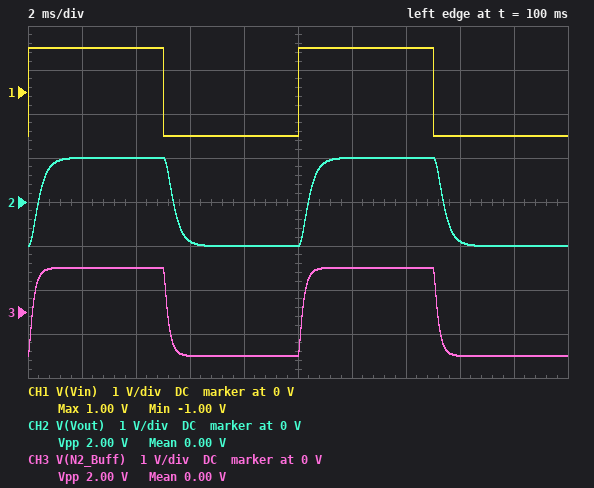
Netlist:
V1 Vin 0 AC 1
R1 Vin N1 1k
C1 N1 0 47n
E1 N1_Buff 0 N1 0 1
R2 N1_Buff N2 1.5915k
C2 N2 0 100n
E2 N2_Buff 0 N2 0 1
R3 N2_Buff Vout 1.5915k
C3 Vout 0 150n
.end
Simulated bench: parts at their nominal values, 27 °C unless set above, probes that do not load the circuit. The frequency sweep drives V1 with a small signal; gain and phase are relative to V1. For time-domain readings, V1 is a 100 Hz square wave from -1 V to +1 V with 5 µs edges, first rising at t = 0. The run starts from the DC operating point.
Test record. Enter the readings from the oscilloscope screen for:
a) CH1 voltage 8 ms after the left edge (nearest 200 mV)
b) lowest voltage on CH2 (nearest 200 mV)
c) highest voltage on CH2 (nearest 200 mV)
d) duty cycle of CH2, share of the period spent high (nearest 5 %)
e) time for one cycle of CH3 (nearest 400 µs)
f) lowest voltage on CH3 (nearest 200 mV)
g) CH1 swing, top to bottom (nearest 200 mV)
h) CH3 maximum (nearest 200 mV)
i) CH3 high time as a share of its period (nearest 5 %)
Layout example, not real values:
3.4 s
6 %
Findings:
-1.0 V
-1.0 V
1.0 V
50 %
10.0 ms
-1.0 V
2.0 V
1.0 V
50 %
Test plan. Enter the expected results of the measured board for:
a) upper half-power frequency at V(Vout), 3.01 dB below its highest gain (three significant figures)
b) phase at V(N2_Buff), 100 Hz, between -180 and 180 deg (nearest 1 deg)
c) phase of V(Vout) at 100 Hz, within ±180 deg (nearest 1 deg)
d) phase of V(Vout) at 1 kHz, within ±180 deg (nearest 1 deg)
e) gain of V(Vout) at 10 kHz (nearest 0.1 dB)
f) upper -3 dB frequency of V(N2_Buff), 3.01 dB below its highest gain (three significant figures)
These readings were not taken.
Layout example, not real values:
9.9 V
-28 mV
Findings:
501 Hz
-7 deg
-16 deg
-118 deg
-53.5 dB
928 Hz
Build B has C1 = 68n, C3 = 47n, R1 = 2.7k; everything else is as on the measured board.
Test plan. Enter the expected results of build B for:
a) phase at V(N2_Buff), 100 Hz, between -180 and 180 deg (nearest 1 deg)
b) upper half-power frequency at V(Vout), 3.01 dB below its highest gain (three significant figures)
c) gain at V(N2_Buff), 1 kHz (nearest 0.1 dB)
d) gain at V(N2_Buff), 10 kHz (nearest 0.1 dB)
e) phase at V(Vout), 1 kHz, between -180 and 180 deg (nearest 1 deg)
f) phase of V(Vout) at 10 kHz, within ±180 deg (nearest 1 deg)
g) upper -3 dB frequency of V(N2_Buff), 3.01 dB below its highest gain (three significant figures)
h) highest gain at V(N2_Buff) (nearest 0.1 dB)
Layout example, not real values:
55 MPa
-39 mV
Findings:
-12 deg
562 Hz
-6.7 dB
-41.3 dB
-119 deg
113 deg
597 Hz
0 dB
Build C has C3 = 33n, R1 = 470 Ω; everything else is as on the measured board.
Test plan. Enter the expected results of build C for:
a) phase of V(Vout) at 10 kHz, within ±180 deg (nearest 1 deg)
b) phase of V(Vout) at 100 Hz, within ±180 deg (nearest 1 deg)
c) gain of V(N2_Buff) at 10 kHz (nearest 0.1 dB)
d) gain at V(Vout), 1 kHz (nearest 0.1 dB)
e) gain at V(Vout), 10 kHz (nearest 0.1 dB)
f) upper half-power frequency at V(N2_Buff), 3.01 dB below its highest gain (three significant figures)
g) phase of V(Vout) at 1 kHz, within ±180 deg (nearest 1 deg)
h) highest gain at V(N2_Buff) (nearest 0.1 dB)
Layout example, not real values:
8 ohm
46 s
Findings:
148 deg
-8 deg
-24.7 dB
-3.5 dB
-35.5 dB
982 Hz
-71 deg
0 dB
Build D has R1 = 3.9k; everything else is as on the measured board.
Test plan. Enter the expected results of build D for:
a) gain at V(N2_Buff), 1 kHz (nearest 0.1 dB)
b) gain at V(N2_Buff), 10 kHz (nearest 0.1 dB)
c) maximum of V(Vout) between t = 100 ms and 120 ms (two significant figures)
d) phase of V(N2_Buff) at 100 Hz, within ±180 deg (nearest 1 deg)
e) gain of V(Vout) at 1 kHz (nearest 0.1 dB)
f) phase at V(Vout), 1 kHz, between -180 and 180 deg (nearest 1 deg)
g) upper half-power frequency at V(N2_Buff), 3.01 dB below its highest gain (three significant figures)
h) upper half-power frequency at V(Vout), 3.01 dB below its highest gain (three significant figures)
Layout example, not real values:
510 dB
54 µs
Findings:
-6.7 dB
-41.3 dB
1.0 V
-12 deg
-11.8 dB
-150 deg
598 Hz
415 Hz
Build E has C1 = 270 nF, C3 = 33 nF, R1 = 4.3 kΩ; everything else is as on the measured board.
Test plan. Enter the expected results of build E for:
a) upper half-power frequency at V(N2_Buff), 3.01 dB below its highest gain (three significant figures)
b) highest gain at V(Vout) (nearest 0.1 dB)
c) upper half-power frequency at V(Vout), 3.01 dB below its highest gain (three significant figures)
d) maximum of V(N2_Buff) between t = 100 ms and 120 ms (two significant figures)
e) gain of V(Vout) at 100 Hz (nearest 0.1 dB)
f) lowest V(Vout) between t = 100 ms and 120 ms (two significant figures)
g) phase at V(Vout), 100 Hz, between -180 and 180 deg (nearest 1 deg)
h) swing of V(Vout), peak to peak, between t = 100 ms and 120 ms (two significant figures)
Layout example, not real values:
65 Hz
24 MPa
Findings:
135 Hz
0 dB
134 Hz
970 mV
-1.9 dB
-970 mV
-44 deg
1.9 V
